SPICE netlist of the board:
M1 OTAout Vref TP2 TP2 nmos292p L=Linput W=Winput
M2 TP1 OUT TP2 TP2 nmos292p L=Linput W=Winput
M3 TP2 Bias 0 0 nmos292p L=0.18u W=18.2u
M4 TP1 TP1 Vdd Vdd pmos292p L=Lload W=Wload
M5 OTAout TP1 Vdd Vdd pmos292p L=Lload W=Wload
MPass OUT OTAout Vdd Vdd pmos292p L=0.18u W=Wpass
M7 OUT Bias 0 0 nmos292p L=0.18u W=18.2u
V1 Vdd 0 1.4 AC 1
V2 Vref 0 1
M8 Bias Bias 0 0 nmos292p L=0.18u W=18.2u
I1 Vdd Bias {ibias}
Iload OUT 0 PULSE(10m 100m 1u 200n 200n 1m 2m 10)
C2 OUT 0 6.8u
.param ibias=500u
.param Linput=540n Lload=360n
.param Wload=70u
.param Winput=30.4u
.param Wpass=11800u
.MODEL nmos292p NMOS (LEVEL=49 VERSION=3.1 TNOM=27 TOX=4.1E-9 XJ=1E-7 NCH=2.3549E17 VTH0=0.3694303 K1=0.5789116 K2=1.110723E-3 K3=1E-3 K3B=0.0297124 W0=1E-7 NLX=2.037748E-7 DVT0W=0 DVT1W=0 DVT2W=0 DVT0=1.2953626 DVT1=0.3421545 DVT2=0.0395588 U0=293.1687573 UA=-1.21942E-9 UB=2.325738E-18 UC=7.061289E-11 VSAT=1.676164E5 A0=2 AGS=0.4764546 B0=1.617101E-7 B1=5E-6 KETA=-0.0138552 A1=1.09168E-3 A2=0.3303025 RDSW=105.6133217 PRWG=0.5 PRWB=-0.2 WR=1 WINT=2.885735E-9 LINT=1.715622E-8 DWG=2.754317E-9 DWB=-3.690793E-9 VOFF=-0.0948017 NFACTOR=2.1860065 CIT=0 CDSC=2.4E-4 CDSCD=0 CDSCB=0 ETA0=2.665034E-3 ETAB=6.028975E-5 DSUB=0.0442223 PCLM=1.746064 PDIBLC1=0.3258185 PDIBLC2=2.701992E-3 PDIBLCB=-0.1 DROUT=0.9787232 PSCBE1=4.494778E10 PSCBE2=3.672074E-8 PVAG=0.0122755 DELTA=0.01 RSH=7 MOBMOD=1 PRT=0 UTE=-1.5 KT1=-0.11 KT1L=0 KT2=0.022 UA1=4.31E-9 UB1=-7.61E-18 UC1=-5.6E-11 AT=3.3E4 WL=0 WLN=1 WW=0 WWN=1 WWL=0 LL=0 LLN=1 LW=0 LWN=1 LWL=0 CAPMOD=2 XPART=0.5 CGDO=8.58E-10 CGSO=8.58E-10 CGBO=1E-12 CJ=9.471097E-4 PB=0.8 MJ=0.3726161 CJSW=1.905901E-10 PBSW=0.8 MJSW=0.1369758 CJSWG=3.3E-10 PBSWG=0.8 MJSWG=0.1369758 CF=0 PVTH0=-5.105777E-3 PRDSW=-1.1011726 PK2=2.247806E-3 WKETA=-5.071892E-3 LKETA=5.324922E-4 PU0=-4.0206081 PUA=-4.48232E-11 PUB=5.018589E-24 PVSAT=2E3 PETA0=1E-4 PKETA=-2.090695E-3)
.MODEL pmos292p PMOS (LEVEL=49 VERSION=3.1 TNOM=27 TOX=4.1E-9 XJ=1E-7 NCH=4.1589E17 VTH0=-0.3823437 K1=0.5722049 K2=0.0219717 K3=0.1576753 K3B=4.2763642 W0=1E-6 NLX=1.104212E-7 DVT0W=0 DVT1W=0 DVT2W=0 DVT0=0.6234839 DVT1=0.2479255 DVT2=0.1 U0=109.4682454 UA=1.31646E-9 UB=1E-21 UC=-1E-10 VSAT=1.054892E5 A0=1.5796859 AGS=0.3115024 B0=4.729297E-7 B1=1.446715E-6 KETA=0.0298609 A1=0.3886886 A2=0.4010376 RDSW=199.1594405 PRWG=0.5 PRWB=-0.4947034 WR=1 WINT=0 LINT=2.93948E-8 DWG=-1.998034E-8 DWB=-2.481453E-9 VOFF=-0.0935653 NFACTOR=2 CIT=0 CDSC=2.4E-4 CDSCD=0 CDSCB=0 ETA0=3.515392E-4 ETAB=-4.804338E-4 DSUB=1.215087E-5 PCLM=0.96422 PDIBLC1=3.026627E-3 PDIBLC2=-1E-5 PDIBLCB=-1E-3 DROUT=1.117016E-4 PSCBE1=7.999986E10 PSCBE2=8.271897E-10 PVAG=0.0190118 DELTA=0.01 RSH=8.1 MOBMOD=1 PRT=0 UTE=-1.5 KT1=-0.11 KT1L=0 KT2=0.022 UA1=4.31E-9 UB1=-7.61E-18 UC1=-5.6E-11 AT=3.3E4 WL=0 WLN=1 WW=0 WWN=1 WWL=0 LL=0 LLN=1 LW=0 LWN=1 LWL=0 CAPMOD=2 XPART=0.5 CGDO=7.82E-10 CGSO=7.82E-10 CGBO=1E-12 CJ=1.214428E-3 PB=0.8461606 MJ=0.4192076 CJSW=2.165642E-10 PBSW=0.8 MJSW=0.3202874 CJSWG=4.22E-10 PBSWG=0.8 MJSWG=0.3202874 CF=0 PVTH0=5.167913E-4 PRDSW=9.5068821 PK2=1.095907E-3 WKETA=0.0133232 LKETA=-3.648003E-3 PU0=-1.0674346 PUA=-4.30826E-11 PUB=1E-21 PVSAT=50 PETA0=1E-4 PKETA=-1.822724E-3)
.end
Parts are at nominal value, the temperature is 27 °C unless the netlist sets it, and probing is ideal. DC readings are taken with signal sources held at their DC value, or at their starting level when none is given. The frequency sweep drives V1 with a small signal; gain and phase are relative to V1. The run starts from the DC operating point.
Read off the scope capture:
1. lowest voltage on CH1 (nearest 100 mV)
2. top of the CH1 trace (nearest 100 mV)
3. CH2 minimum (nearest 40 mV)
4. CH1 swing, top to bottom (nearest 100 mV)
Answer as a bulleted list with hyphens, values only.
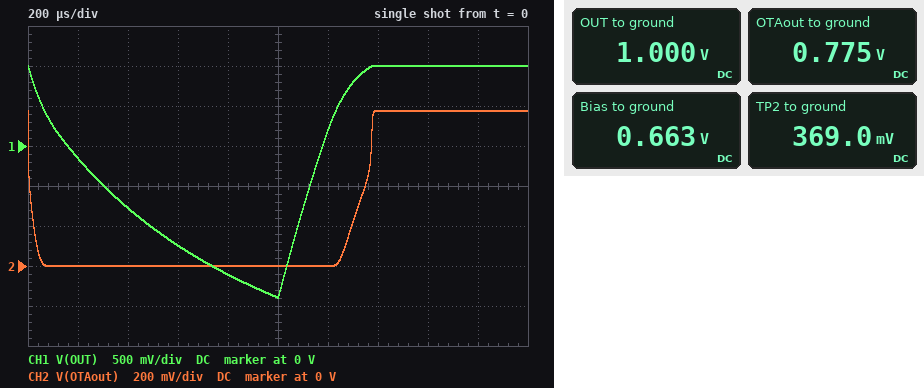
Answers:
- -1.9 V
- 1.0 V
- 0 V
- 2.9 V
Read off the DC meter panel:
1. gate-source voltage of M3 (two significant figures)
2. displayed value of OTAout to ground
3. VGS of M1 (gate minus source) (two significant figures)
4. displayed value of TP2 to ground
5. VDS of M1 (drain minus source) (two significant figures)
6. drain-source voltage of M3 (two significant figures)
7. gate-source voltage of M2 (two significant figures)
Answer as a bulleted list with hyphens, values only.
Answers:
- 660 mV
- 0.775 V
- 630 mV
- 369.0 mV
- 410 mV
- 370 mV
- 630 mV
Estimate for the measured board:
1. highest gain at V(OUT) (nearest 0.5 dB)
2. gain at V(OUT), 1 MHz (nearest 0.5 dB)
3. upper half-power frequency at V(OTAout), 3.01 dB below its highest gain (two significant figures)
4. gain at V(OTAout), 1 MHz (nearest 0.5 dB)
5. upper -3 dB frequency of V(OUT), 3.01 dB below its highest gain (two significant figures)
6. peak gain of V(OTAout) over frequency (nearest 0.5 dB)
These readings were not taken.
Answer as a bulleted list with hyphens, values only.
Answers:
- -56.0 dB
- -64.5 dB
- 650 kHz
- -3.5 dB
- 450 kHz
- 0.5 dB
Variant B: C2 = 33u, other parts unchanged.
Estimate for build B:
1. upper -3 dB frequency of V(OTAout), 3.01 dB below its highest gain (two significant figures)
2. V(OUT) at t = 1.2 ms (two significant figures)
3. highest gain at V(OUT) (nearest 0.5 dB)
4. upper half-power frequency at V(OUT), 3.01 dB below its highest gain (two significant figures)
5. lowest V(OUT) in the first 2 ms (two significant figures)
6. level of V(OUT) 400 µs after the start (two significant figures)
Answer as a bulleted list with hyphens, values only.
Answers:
- 680 kHz
- 200 mV
- -60.0 dB
- 14 kHz
- -180 mV
- 340 mV
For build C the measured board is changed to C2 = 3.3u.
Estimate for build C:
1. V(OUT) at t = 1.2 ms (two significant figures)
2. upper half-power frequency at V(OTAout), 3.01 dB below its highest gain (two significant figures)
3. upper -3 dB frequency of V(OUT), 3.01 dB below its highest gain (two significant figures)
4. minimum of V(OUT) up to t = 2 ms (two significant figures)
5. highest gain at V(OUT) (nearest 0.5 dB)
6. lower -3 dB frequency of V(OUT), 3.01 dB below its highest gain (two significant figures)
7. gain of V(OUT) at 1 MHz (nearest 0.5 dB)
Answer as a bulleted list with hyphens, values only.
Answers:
- 930 mV
- 590 kHz
- 510 kHz
- -2.7 V
- -50.0 dB
- 87 kHz
- -58.0 dB
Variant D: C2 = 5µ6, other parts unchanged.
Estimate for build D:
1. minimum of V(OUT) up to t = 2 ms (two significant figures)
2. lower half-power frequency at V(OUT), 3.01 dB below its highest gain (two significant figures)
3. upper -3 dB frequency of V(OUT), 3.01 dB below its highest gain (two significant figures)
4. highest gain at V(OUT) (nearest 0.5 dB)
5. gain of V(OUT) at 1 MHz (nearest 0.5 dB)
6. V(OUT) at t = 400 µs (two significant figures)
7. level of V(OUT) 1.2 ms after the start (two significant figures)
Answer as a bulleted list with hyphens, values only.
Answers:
- -2.1 V
- 41 kHz
- 470 kHz
- -54.5 dB
- -62.5 dB
- -990 mV
- 370 mV
